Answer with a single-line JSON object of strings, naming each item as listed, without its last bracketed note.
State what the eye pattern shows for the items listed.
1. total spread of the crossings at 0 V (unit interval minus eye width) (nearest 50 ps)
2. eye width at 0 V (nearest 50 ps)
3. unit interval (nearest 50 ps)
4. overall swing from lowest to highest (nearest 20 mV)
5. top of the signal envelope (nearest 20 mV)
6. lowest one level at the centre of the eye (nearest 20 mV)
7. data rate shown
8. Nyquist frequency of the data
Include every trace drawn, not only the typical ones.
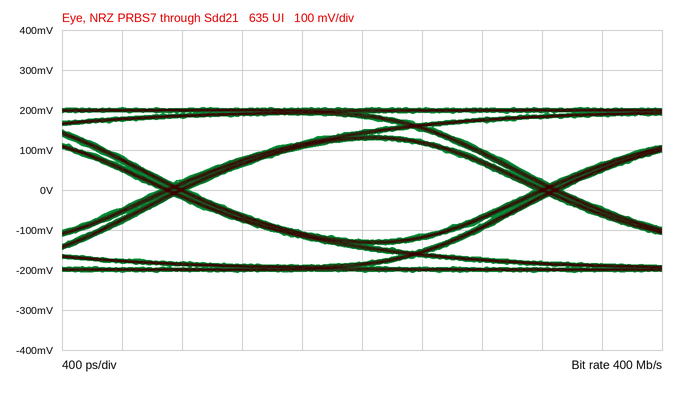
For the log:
{"total spread of the crossings at 0 V (unit interval minus eye width)": "200 ps", "eye width at 0 V": "2.30 ns", "unit interval": "2.50 ns", "overall swing from lowest to highest": "420 mV", "top of the signal envelope": "200 mV", "lowest one level at the centre of the eye": "120 mV", "data rate shown": "400 Mb/s", "Nyquist frequency of the data": "200 MHz"}
